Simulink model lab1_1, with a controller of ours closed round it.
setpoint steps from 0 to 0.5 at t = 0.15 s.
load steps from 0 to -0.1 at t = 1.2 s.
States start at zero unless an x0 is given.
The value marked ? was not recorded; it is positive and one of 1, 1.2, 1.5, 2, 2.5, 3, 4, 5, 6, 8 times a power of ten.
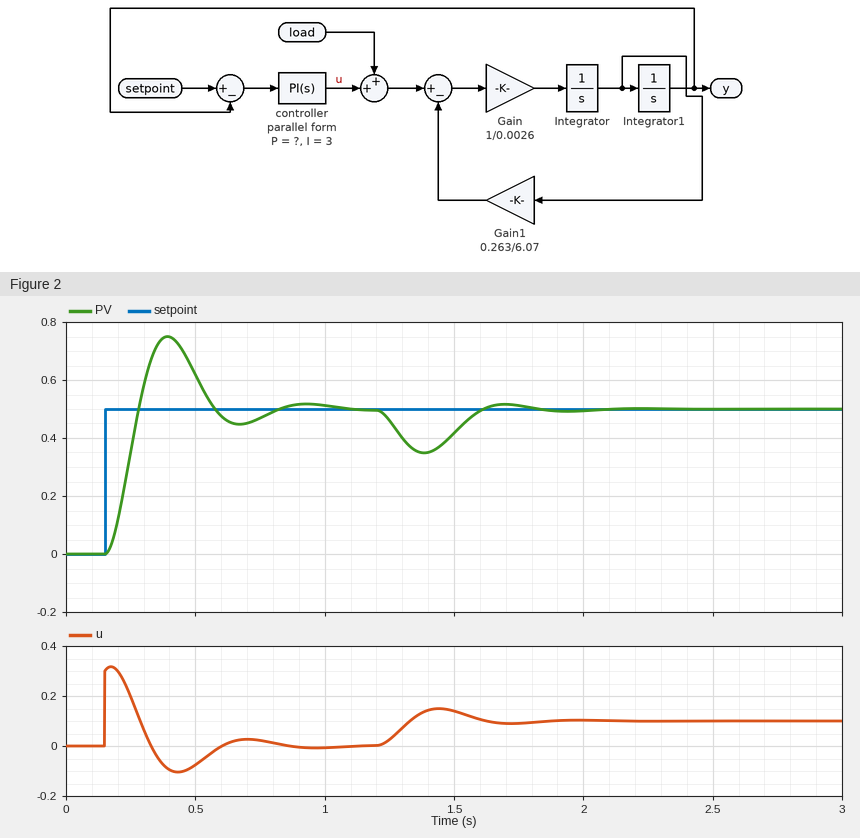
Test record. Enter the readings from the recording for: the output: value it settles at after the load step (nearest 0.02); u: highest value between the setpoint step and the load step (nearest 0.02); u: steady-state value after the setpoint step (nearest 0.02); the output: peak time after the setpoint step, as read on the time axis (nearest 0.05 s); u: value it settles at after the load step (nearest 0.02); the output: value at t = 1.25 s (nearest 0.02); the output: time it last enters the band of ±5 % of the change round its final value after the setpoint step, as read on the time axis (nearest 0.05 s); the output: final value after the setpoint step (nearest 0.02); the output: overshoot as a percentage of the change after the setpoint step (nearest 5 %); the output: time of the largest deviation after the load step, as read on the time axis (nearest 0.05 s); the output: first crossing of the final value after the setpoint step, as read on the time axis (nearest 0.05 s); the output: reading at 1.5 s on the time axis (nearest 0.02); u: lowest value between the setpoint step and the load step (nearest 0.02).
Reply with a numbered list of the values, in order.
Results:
1. 0.50
2. 0.32
3. 0.00
4. 0.40 s
5. 0.10
6. 0.46
7. 0.75 s
8. 0.50
9. 50 %
10. 1.40 s
11. 0.30 s
12. 0.42
13. -0.10
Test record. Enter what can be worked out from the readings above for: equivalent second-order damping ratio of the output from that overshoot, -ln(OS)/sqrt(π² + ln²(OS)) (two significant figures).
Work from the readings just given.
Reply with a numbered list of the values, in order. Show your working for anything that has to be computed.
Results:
1. ln(0.5) = -0.693; 0.693 / sqrt(9.870 + 0.480) = 0.22
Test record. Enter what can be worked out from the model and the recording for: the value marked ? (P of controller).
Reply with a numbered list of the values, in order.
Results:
1. 0.6
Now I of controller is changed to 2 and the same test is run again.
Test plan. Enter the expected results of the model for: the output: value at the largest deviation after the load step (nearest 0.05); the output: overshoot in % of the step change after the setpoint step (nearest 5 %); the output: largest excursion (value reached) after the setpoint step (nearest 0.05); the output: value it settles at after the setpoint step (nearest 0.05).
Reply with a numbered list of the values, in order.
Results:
1. 0.35
2. 40 %
3. 0.70
4. 0.50
